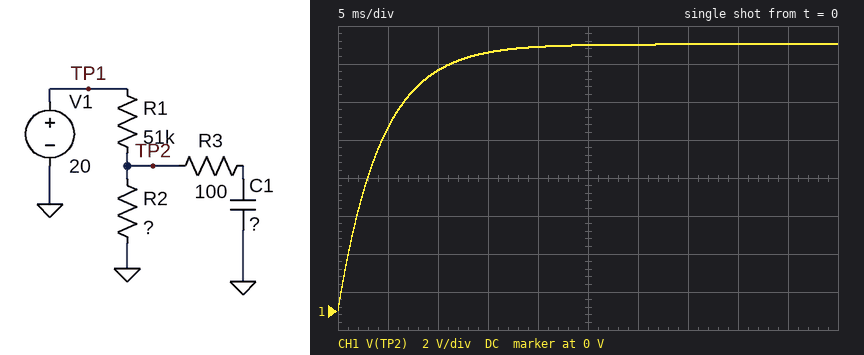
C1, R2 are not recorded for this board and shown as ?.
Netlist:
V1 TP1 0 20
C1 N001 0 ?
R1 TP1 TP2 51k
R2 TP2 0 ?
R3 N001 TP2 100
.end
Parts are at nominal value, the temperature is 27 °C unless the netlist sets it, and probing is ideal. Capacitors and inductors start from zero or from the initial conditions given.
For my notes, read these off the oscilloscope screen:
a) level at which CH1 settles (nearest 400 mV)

14.0 V
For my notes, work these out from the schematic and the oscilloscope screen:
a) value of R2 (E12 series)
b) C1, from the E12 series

120 kΩ
120 nF
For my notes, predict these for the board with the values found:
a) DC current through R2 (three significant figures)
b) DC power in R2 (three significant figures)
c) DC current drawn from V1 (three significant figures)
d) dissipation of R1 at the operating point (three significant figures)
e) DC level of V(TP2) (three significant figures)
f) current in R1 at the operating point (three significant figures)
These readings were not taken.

117 µA
1.64 mW
117 µA
698 µW
14.0 V
117 µA
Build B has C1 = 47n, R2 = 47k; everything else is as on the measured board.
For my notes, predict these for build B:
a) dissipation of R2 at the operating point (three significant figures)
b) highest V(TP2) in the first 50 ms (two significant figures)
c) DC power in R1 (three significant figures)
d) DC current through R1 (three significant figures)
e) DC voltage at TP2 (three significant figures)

1.96 mW
9.6 V
2.12 mW
204 µA
9.59 V
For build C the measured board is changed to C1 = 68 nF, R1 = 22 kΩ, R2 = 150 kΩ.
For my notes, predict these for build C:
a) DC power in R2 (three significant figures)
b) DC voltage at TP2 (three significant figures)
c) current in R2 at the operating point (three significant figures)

2.03 mW
17.4 V
116 µA
